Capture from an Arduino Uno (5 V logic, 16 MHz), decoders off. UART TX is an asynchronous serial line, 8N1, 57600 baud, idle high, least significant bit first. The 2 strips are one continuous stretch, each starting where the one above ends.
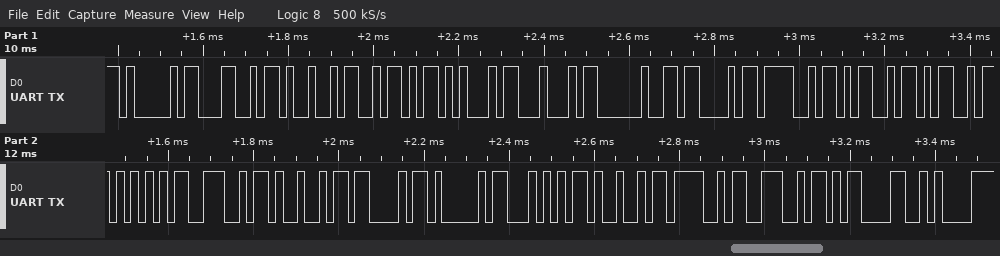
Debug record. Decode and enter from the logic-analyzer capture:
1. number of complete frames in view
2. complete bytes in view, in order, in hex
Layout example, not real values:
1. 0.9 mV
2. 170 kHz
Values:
1. 22
2. 41 4C 49 5A 45 44 20 43 4F 4D 4D 55 4E 49 43 41 54 49 4F 4E 0D 0A
